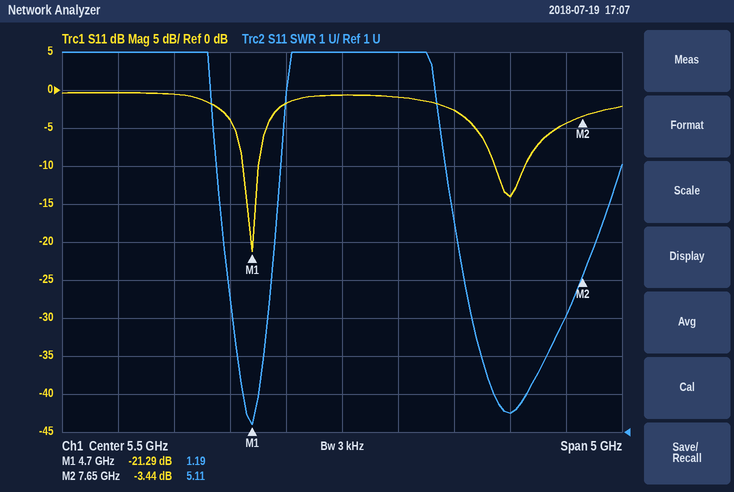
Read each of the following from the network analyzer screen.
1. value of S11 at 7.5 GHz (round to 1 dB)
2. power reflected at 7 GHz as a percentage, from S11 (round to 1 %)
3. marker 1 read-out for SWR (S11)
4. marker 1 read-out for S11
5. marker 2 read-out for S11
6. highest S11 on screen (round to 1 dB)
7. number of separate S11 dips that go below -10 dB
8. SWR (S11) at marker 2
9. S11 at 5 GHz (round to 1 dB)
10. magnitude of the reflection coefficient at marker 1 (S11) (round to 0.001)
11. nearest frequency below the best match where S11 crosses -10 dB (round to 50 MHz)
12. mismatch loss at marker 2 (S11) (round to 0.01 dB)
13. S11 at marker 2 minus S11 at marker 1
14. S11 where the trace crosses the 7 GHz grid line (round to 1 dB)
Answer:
-4 dB
4 %
1.19
-21.29 dB
-3.44 dB
0 dB
2
5.11
-2 dB
0.086
4.60 GHz
2.62 dB
17.85 dB
-14 dB
